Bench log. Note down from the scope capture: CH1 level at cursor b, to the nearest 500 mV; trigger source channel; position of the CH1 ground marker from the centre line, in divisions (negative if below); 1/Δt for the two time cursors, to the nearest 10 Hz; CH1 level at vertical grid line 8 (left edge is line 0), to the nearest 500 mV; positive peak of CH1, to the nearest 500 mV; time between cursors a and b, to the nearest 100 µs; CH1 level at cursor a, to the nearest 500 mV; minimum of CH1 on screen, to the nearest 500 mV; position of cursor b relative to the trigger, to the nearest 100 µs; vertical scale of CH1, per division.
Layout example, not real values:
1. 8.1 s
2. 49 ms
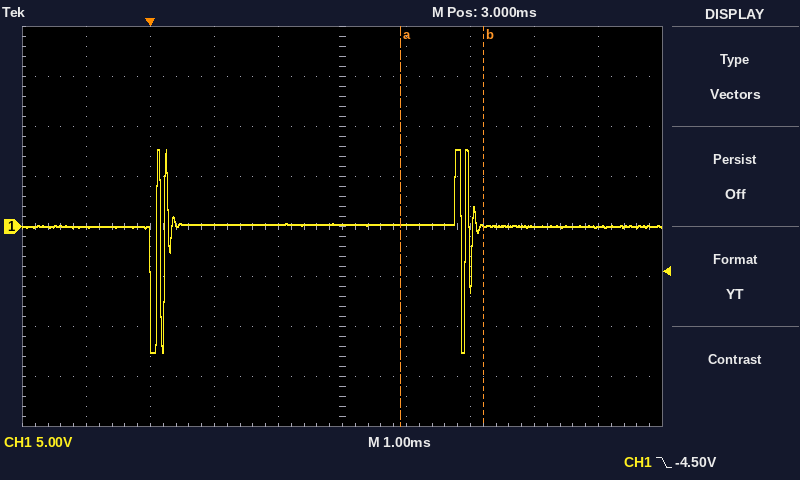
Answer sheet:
1. 0.0 V
2. CH1
3. 0.0 div
4. 770 Hz
5. 0.0 V
6. 7.5 V
7. 1.3 ms
8. 0.0 V
9. -12.5 V
10. +5.2 ms
11. 5 V
